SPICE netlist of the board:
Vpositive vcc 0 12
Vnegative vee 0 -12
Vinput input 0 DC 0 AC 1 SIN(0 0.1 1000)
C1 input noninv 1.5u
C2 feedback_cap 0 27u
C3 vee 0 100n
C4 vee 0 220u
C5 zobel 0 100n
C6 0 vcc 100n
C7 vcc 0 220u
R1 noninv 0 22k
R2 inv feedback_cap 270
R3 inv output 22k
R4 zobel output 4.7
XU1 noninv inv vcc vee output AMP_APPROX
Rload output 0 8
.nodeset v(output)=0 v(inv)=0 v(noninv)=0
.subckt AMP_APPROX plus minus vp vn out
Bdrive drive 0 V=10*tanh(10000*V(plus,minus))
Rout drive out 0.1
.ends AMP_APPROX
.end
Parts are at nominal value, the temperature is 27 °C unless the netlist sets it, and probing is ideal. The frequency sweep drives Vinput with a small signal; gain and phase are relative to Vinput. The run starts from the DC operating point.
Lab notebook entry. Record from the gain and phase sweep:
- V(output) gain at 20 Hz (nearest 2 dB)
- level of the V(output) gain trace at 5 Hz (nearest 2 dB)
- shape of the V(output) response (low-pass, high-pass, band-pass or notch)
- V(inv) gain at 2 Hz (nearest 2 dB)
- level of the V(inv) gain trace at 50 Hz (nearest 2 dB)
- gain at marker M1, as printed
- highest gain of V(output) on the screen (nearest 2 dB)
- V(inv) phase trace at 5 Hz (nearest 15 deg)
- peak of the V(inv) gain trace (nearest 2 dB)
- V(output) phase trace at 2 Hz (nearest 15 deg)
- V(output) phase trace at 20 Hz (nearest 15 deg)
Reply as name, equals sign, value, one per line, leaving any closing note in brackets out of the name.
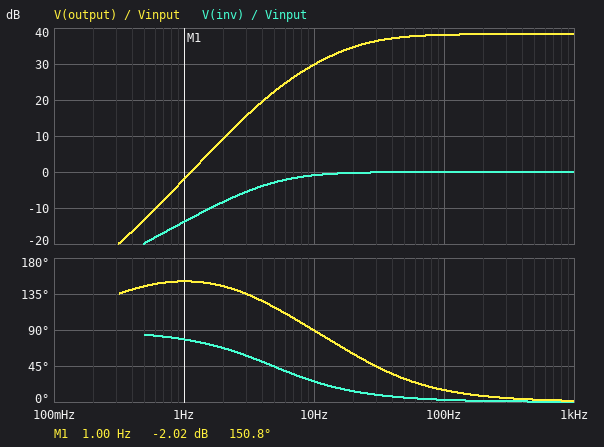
V(output) gain at 20 Hz = 34 dB
level of the V(output) gain trace at 5 Hz = 22 dB
shape of the V(output) response = high-pass
V(inv) gain at 2 Hz = -8 dB
level of the V(inv) gain trace at 50 Hz = 0 dB
gain at marker M1, as printed = -2.02 dB
highest gain of V(output) on the screen = 38 dB
V(inv) phase trace at 5 Hz = 45 deg
peak of the V(inv) gain trace = 0 dB
V(output) phase trace at 2 Hz = 150 deg
V(output) phase trace at 20 Hz = 60 deg
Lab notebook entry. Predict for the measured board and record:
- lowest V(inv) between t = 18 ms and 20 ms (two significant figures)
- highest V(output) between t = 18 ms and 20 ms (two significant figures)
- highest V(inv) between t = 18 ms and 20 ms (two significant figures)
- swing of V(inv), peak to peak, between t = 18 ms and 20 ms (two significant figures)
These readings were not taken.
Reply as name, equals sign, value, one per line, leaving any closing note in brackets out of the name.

lowest V(inv) between t = 18 ms and 20 ms = -100 mV
highest V(output) between t = 18 ms and 20 ms = 8.2 V
highest V(inv) between t = 18 ms and 20 ms = 100 mV
swing of V(inv), peak to peak, between t = 18 ms and 20 ms = 200 mV
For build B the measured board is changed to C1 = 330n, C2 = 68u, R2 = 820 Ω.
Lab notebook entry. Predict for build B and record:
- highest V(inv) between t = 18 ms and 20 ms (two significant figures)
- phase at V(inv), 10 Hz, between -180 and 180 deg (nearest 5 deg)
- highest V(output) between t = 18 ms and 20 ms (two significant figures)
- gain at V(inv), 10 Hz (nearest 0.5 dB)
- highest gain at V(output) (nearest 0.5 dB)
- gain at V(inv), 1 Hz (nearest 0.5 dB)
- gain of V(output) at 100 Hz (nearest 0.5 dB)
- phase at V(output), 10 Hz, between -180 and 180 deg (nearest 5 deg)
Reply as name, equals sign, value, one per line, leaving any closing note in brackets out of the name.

highest V(inv) between t = 18 ms and 20 ms = 100 mV
phase at V(inv), 10 Hz, between -180 and 180 deg = 65 deg
highest V(output) between t = 18 ms and 20 ms = 2.8 V
gain at V(inv), 10 Hz = -7.5 dB
highest gain at V(output) = 29.0 dB
gain at V(inv), 1 Hz = -27.0 dB
gain of V(output) at 100 Hz = 28.5 dB
phase at V(output), 10 Hz, between -180 and 180 deg = 80 deg
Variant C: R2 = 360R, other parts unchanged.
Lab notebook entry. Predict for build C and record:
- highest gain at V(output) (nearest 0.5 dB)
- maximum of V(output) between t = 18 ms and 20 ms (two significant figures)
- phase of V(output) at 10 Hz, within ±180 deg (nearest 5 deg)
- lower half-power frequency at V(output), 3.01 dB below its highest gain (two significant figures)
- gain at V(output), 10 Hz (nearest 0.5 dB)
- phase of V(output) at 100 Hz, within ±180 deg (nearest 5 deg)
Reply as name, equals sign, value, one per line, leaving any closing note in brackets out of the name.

highest gain at V(output) = 36.0 dB
maximum of V(output) between t = 18 ms and 20 ms = 6.2 V
phase of V(output) at 10 Hz, within ±180 deg = 85 deg
lower half-power frequency at V(output), 3.01 dB below its highest gain = 18 Hz
gain at V(output), 10 Hz = 29.5 dB
phase of V(output) at 100 Hz, within ±180 deg = 10 deg
